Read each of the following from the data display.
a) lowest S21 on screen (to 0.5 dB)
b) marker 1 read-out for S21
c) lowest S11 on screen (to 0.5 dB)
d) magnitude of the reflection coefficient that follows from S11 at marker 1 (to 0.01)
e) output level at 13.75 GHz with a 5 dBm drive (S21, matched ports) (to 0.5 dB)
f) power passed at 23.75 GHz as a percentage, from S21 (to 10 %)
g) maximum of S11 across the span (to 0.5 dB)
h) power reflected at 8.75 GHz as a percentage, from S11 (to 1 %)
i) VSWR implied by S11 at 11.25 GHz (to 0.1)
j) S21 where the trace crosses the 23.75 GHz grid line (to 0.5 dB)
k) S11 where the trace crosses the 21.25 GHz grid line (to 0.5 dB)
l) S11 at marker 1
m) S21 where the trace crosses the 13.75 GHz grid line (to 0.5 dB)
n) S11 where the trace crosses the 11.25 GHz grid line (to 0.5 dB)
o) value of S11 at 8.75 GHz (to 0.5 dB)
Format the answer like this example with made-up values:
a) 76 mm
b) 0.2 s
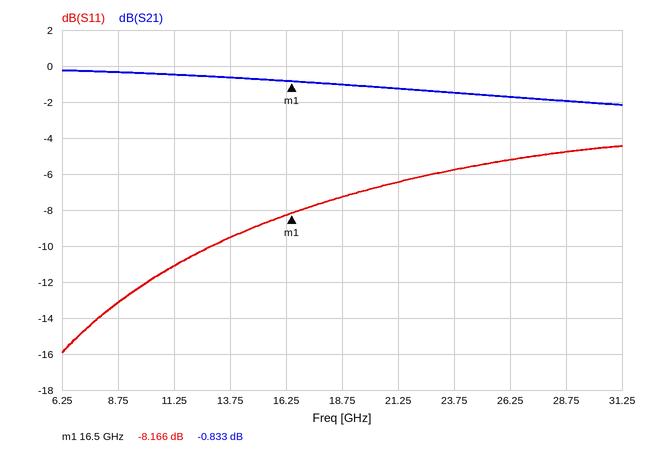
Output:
a) -2.0 dB
b) -0.833 dB
c) -16.0 dB
d) 0.39
e) 4.5 dBm
f) 70 %
g) -4.5 dB
h) 5 %
i) 1.8
j) -1.5 dB
k) -6.5 dB
l) -8.166 dB
m) -0.5 dB
n) -11.0 dB
o) -13.0 dB
